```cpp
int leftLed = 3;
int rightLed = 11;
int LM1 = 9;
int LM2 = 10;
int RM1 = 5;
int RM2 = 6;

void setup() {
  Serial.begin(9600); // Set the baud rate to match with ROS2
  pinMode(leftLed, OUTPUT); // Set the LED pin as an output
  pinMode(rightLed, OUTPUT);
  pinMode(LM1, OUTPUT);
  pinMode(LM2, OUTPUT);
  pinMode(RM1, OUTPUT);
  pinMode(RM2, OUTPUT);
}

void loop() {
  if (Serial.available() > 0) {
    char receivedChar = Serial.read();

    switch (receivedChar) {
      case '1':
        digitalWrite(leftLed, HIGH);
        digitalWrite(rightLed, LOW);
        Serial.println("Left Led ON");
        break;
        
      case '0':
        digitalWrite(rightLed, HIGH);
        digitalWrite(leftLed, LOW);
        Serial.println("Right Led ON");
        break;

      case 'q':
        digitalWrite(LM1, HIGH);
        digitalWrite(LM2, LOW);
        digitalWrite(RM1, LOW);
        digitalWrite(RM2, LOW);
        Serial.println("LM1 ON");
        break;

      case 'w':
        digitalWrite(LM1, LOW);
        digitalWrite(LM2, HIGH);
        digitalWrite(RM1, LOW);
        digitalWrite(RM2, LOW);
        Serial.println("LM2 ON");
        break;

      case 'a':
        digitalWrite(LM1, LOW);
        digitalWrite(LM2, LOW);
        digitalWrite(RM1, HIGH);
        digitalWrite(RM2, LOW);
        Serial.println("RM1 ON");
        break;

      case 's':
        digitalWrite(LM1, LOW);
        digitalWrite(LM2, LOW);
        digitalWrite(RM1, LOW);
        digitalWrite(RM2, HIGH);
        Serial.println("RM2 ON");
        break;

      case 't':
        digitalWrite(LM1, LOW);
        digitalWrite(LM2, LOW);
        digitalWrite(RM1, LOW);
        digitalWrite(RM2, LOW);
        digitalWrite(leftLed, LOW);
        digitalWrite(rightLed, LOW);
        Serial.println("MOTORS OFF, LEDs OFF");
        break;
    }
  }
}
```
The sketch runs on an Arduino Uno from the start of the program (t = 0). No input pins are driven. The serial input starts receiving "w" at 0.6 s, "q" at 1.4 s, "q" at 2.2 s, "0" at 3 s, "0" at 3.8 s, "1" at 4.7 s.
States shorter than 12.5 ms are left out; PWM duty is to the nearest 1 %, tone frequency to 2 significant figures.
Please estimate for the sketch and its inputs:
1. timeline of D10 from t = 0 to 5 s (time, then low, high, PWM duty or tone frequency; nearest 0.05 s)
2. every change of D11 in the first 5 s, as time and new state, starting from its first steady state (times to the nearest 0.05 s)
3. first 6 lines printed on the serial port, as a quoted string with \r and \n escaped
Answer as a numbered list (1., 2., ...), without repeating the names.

1. 0 s low; 0.6 s high; 1.4 s low
2. 0 s low; 3 s high; 4.7 s low
3. "LM2 ON\r\nLM1 ON\r\nLM1 ON\r\nRight Led ON\r\nRight Led ON\r\nLeft Led ON\r\n"
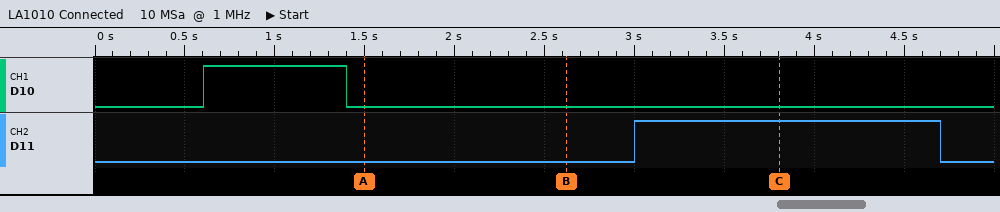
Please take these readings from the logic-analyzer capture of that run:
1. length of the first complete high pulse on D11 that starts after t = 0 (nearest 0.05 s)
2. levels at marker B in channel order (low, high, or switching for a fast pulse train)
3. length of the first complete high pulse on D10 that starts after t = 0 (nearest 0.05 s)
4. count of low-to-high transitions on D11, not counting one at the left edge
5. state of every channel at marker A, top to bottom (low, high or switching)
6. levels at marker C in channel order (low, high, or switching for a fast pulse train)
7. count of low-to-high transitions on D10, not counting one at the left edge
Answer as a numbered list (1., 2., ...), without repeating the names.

1. 1.70 s
2. D10 low, D11 low
3. 0.80 s
4. 1
5. D10 low, D11 low
6. D10 low, D11 high
7. 1
